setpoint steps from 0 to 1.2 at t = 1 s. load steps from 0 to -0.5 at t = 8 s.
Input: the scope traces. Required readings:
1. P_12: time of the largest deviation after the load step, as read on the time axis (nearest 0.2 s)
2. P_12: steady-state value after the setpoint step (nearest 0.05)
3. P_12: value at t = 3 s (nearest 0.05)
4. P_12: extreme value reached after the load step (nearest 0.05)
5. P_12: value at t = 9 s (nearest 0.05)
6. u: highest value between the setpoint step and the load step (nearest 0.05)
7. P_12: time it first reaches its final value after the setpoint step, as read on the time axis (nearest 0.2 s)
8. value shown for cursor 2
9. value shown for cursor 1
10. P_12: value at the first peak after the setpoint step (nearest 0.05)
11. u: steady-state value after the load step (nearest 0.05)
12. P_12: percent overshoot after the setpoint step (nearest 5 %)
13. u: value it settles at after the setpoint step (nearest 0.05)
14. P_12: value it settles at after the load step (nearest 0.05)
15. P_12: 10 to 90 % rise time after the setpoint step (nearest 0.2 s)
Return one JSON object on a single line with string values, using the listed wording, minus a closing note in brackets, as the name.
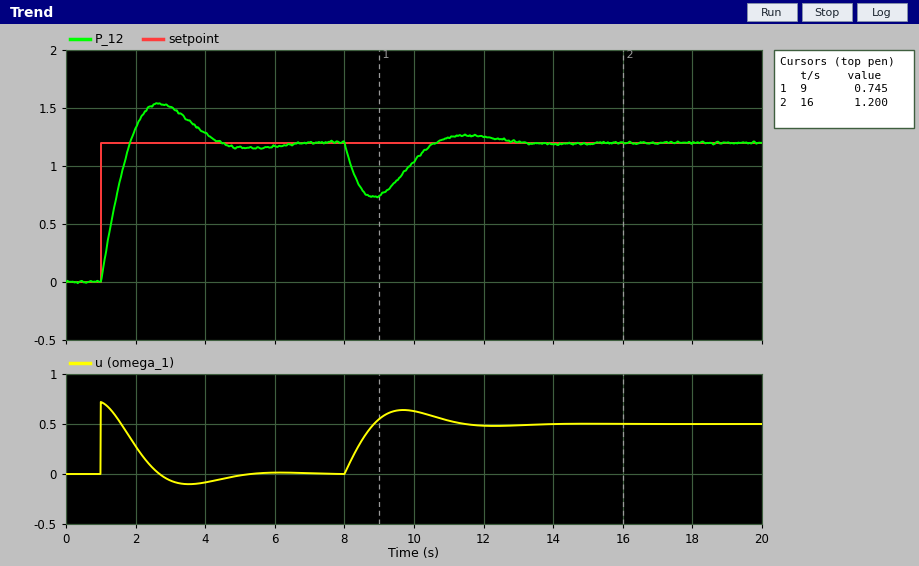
{"P_12: time of the largest deviation after the load step, as read on the time axis": "8.8 s", "P_12: steady-state value after the setpoint step": "1.20", "P_12: value at t = 3 s": "1.50", "P_12: extreme value reached after the load step": "0.75", "P_12: value at t = 9 s": "0.75", "u: highest value between the setpoint step and the load step": "0.70", "P_12: time it first reaches its final value after the setpoint step, as read on the time axis": "1.8 s", "value shown for cursor 2": "1.200", "value shown for cursor 1": "0.745", "P_12: value at the first peak after the setpoint step": "1.55", "u: steady-state value after the load step": "0.50", "P_12: percent overshoot after the setpoint step": "30 %", "u: value it settles at after the setpoint step": "0.00", "P_12: value it settles at after the load step": "1.20", "P_12: 10 to 90 % rise time after the setpoint step": "0.6 s"}
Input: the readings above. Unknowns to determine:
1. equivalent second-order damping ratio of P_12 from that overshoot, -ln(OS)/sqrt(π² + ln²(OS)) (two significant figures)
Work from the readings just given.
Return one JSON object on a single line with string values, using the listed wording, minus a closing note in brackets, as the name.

{"equivalent second-order damping ratio of P_12 from that overshoot, -ln(OS)/sqrt(π² + ln²(OS))": "0.36"}
